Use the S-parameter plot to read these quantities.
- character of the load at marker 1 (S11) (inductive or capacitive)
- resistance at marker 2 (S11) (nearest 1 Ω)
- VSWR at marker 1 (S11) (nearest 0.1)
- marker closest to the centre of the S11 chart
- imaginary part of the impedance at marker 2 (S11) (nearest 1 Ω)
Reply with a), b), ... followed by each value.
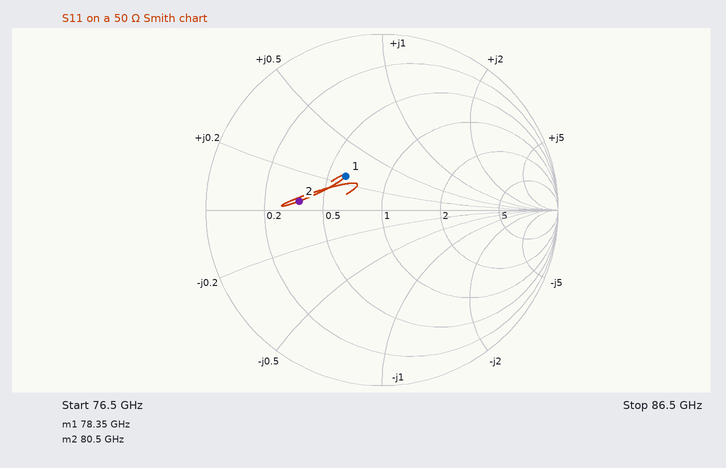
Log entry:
a) inductive
b) 18 Ω
c) 1.8
d) marker 1
e) +2 Ω
